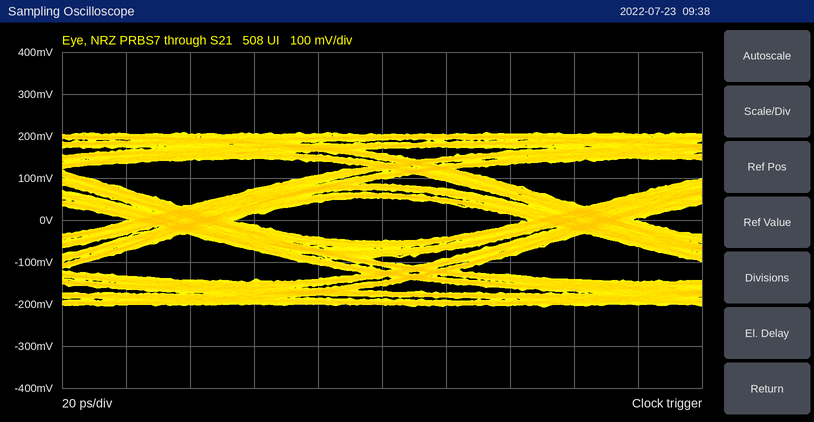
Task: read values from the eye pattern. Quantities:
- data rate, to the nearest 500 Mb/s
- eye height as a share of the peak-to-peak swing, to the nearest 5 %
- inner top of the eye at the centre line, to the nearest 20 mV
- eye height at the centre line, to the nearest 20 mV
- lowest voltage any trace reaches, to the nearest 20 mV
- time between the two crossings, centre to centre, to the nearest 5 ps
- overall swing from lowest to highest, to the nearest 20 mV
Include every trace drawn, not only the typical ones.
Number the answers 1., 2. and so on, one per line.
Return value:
1. 8.0 Gb/s
2. 25 %
3. 60 mV
4. 100 mV
5. -200 mV
6. 125 ps
7. 420 mV
